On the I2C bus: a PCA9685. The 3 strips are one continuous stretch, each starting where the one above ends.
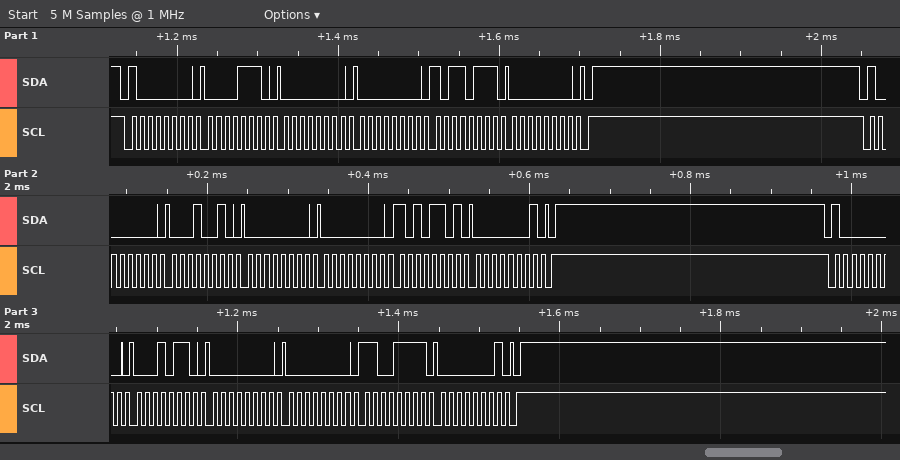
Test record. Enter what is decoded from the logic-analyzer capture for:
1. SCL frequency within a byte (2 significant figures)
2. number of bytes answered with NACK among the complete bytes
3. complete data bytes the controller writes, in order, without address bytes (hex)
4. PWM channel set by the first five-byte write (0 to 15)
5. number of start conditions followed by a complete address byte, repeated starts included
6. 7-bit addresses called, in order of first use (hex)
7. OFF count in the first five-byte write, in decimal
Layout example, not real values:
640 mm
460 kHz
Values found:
100 kHz
0
0E 00 00 B7 00 12 00 00 AD 01 16 00 00 CF 01
2
3
0x40
183
